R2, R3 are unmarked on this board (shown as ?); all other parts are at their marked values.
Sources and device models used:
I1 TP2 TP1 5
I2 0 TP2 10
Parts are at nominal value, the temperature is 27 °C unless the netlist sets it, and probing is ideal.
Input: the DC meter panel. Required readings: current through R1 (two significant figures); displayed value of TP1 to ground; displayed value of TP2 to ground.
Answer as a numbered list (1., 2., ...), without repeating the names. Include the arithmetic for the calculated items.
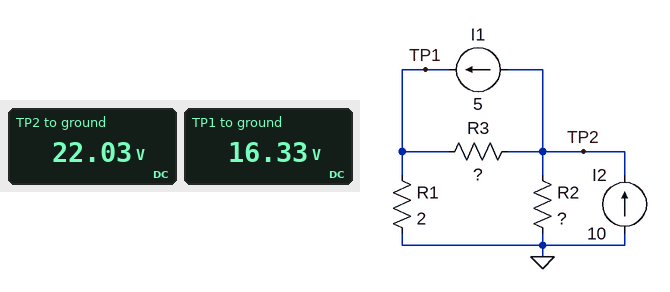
1. (16.33 V) / 2 Ω = 8.2 A
2. 16.33 V
3. 22.03 V
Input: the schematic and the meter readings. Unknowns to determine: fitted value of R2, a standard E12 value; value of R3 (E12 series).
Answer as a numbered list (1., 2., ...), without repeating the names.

1. 12 Ω
2. 1.8 Ω
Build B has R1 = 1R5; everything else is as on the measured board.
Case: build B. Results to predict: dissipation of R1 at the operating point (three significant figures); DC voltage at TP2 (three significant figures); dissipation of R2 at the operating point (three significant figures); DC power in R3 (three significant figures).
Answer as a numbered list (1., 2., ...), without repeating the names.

1. 107 W
2. 18.8 V
3. 29.5 W
4. 21.2 W
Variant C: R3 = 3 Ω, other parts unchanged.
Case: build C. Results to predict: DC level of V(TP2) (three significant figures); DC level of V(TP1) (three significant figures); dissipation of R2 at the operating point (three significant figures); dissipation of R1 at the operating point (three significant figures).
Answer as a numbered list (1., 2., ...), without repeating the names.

1. 24.7 V
2. 15.9 V
3. 50.9 W
4. 126 W
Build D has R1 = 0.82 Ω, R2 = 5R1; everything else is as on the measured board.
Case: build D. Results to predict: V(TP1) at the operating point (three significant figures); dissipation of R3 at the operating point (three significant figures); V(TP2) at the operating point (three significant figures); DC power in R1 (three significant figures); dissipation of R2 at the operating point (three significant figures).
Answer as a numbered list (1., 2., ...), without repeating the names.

1. 6.37 V
2. 13.8 W
3. 11.4 V
4. 49.5 W
5. 25.3 W
